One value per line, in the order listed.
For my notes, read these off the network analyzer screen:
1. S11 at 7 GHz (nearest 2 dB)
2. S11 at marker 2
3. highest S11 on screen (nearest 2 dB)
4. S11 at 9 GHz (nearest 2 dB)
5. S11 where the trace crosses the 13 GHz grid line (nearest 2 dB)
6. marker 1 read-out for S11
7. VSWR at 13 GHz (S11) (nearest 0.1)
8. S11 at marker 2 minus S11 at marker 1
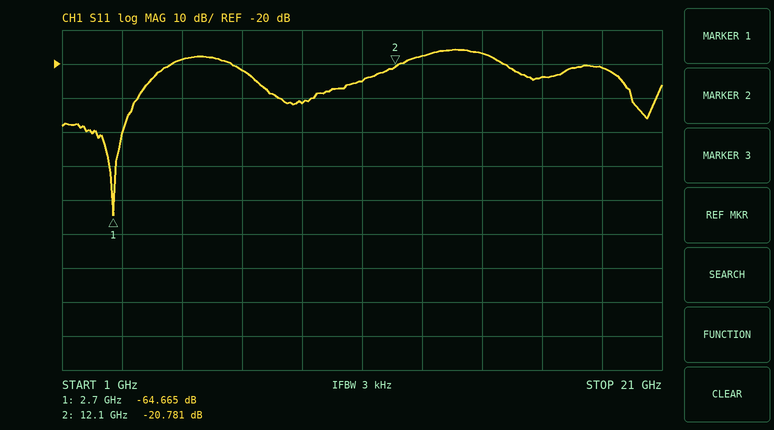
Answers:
-22 dB
-20.781 dB
-16 dB
-32 dB
-18 dB
-64.665 dB
1.3
43.884 dB
